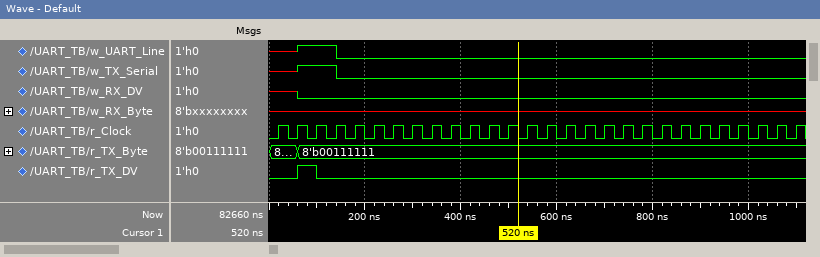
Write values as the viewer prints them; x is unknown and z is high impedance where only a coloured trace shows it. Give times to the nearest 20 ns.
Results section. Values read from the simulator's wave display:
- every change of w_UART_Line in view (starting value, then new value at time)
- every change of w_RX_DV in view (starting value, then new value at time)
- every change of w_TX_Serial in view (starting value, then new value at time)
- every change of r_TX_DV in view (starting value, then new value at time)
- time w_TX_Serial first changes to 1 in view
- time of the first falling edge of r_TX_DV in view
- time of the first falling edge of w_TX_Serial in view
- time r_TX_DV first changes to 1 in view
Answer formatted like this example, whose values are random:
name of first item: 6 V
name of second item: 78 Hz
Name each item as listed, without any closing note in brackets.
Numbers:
every change of w_UART_Line in view: x, 1 at 60 ns, 0 at 140 ns
every change of w_RX_DV in view: x, 0 at 60 ns
every change of w_TX_Serial in view: x, 1 at 60 ns, 0 at 140 ns
every change of r_TX_DV in view: 0, 1 at 60 ns, 0 at 100 ns
time w_TX_Serial first changes to 1 in view: 60 ns
time of the first falling edge of r_TX_DV in view: 100 ns
time of the first falling edge of w_TX_Serial in view: 140 ns
time r_TX_DV first changes to 1 in view: 60 ns
